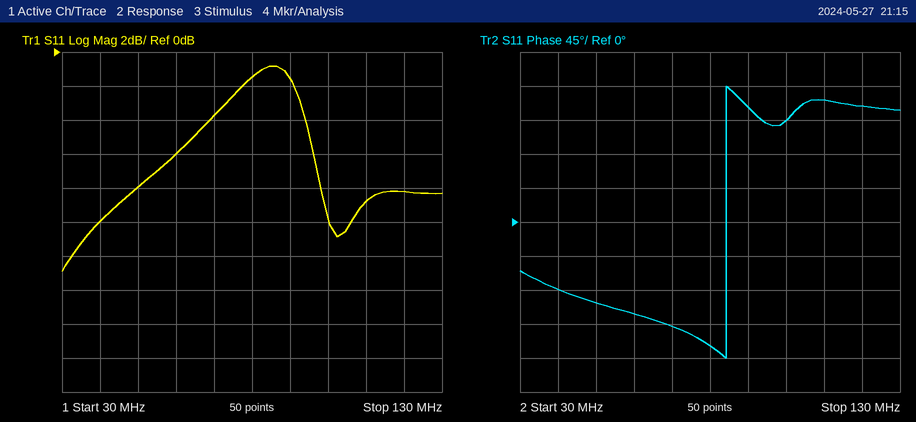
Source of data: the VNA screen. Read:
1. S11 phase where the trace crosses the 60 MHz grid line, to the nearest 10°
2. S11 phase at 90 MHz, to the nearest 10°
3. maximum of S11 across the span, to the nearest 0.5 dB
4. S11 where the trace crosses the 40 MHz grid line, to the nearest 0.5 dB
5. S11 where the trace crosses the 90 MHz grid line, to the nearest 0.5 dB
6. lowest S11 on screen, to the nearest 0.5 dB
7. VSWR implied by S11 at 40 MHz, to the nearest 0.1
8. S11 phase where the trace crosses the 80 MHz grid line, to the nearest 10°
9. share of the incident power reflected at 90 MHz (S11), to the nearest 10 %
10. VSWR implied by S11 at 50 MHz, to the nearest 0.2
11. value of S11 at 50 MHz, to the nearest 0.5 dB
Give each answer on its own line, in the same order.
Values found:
-120°
150°
-1.0 dB
-10.0 dB
-1.5 dB
-13.0 dB
1.9
-160°
70 %
2.4
-8.0 dB
